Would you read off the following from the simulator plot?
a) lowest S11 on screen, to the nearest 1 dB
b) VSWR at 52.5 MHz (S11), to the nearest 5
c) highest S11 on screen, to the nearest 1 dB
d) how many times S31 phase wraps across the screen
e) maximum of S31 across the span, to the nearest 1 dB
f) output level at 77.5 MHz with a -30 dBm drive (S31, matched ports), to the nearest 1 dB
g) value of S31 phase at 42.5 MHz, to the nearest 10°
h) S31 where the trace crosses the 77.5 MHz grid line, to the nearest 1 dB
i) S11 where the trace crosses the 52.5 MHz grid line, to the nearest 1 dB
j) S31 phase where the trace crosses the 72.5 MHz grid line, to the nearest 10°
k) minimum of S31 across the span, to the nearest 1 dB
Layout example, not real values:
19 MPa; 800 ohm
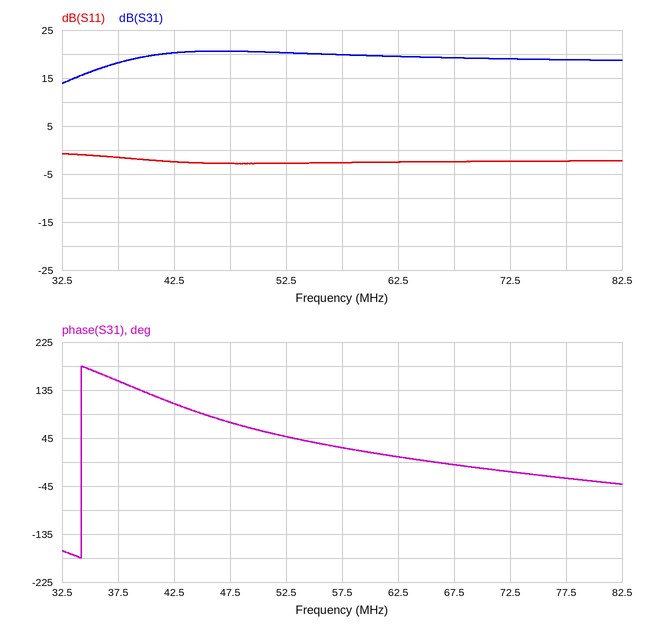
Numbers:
-3 dB; 5; -1 dB; 1; 21 dB; -11 dBm; 110°; 19 dB; -3 dB; -20°; 14 dB
